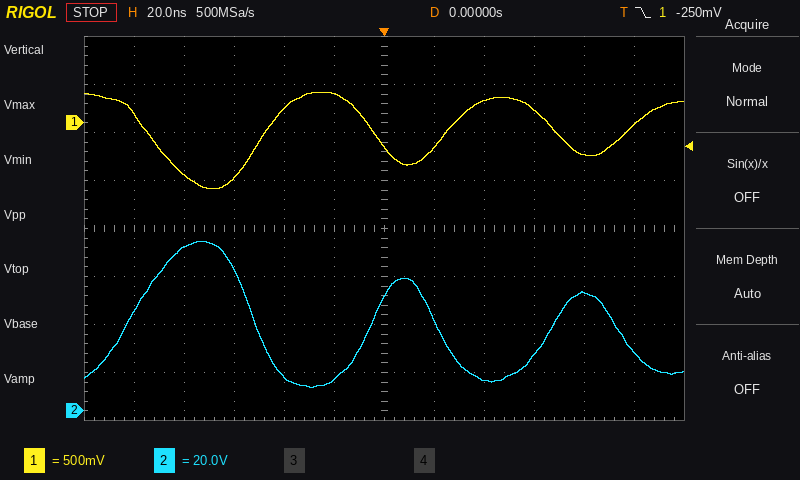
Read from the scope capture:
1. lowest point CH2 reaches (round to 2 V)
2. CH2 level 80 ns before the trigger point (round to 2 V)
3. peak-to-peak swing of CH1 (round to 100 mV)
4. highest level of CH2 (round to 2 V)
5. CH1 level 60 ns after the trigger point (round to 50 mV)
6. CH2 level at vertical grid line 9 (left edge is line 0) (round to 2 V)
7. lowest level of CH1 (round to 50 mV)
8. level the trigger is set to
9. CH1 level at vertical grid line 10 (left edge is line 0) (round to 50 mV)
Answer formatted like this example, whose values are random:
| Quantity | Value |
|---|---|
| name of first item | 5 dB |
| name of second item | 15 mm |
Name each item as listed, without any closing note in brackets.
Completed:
| Quantity | Value |
|---|---|
| lowest point CH2 reaches | 10 V |
| CH2 level 80 ns before the trigger point | 68 V |
| peak-to-peak swing of CH1 | 1.00 V |
| highest level of CH2 | 70 V |
| CH1 level 60 ns after the trigger point | 150 mV |
| CH2 level at vertical grid line 9 (left edge is line 0) | 24 V |
| lowest level of CH1 | -700 mV |
| level the trigger is set to | -250 mV |
| CH1 level at vertical grid line 10 (left edge is line 0) | -350 mV |
